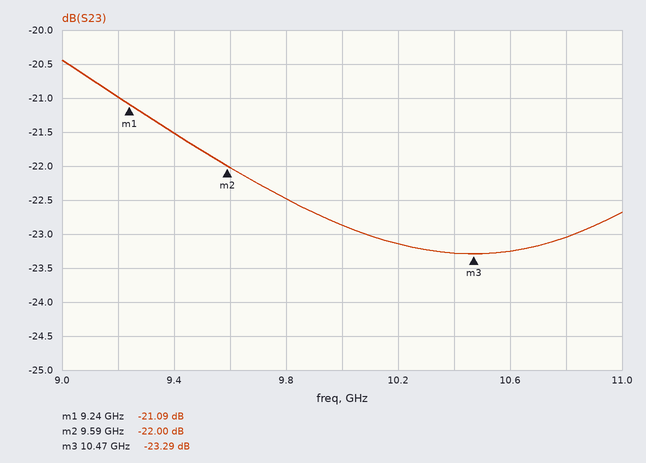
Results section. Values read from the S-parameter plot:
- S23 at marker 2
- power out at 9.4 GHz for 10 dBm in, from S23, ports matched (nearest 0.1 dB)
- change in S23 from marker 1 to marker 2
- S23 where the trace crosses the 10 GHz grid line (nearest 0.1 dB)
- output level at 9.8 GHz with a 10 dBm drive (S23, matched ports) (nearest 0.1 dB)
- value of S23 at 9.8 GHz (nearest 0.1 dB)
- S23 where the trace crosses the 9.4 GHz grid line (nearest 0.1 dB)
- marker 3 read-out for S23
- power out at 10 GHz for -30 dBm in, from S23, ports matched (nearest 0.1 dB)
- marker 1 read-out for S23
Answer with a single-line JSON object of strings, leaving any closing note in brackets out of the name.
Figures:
{"S23 at marker 2": "-22.00 dB", "power out at 9.4 GHz for 10 dBm in, from S23, ports matched": "-11.5 dBm", "change in S23 from marker 1 to marker 2": "-0.91 dB", "S23 where the trace crosses the 10 GHz grid line": "-22.9 dB", "output level at 9.8 GHz with a 10 dBm drive (S23, matched ports)": "-12.5 dBm", "value of S23 at 9.8 GHz": "-22.5 dB", "S23 where the trace crosses the 9.4 GHz grid line": "-21.5 dB", "marker 3 read-out for S23": "-23.29 dB", "power out at 10 GHz for -30 dBm in, from S23, ports matched": "-52.9 dBm", "marker 1 read-out for S23": "-21.09 dB"}
